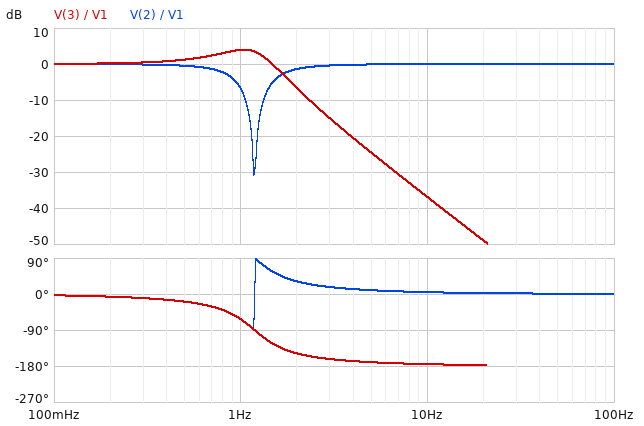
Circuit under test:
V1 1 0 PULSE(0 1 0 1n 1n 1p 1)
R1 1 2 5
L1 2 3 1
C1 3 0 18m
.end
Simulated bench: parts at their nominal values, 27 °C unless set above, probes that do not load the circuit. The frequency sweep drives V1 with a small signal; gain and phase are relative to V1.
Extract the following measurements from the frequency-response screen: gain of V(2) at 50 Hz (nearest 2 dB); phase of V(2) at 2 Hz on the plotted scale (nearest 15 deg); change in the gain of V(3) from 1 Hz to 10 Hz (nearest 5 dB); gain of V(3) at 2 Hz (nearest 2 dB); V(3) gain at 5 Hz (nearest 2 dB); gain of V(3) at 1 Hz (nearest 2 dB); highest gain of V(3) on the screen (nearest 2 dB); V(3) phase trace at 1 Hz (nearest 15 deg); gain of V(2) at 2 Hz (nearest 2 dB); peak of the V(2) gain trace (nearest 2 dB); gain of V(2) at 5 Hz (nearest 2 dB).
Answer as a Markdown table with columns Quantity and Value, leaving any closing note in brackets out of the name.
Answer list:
| Quantity | Value |
|---|---|
| gain of V(2) at 50 Hz | 0 dB |
| phase of V(2) at 2 Hz on the plotted scale | 30 deg |
| change in the gain of V(3) from 1 Hz to 10 Hz | -40 dB |
| gain of V(3) at 2 Hz | -6 dB |
| V(3) gain at 5 Hz | -24 dB |
| gain of V(3) at 1 Hz | 4 dB |
| highest gain of V(3) on the screen | 4 dB |
| V(3) phase trace at 1 Hz | -60 deg |
| gain of V(2) at 2 Hz | -2 dB |
| peak of the V(2) gain trace | 0 dB |
| gain of V(2) at 5 Hz | 0 dB |
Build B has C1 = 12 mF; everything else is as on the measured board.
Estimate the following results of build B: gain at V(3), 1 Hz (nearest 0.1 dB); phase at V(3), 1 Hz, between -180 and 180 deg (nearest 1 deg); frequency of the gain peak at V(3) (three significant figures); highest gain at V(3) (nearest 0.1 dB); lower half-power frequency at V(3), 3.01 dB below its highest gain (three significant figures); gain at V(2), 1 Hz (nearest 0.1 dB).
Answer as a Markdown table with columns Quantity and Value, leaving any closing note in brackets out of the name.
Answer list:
| Quantity | Value |
|---|---|
| gain at V(3), 1 Hz | 3.8 dB |
| phase at V(3), 1 Hz, between -180 and 180 deg | -36 deg |
| frequency of the gain peak at V(3) | 1.34 Hz |
| highest gain at V(3) | 5.6 dB |
| lower half-power frequency at V(3), 3.01 dB below its highest gain | 826 mHz |
| gain at V(2), 1 Hz | -1.8 dB |
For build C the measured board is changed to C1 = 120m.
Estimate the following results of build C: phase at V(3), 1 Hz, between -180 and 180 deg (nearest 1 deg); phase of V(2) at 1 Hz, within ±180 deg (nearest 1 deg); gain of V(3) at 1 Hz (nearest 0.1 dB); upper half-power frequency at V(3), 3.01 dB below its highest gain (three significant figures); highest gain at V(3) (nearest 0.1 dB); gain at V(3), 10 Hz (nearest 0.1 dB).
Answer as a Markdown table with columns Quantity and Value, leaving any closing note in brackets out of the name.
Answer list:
| Quantity | Value |
|---|---|
| phase at V(3), 1 Hz, between -180 and 180 deg | -135 deg |
| phase of V(2) at 1 Hz, within ±180 deg | 45 deg |
| gain of V(3) at 1 Hz | -14.5 dB |
| upper half-power frequency at V(3), 3.01 dB below its highest gain | 361 mHz |
| highest gain at V(3) | 0 dB |
| gain at V(3), 10 Hz | -53.5 dB |
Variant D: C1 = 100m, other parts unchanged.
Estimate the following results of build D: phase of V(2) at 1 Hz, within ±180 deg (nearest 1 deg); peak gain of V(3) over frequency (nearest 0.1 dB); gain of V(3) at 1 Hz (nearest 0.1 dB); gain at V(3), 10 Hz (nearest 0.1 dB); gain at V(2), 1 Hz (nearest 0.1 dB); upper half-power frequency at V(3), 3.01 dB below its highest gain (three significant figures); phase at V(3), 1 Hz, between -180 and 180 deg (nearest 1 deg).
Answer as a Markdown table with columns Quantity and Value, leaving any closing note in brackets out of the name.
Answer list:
| Quantity | Value |
|---|---|
| phase of V(2) at 1 Hz, within ±180 deg | 47 deg |
| peak gain of V(3) over frequency | 0 dB |
| gain of V(3) at 1 Hz | -12.7 dB |
| gain at V(3), 10 Hz | -51.9 dB |
| gain at V(2), 1 Hz | -3.3 dB |
| upper half-power frequency at V(3), 3.01 dB below its highest gain | 445 mHz |
| phase at V(3), 1 Hz, between -180 and 180 deg | -133 deg |
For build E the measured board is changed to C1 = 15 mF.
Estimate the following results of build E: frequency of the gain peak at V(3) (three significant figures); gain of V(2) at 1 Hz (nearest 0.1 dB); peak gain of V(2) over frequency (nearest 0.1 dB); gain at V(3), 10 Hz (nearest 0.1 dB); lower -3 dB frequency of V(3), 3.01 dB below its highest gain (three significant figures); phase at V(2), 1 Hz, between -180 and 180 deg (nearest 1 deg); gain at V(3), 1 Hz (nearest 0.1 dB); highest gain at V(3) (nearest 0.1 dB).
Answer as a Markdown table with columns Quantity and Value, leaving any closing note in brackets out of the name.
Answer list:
| Quantity | Value |
|---|---|
| frequency of the gain peak at V(3) | 1.17 Hz |
| gain of V(2) at 1 Hz | -3.7 dB |
| peak gain of V(2) over frequency | 0 dB |
| gain at V(3), 10 Hz | -35.3 dB |
| lower -3 dB frequency of V(3), 3.01 dB below its highest gain | 623 mHz |
| phase at V(2), 1 Hz, between -180 and 180 deg | -49 deg |
| gain at V(3), 1 Hz | 4.1 dB |
| highest gain at V(3) | 4.7 dB |
